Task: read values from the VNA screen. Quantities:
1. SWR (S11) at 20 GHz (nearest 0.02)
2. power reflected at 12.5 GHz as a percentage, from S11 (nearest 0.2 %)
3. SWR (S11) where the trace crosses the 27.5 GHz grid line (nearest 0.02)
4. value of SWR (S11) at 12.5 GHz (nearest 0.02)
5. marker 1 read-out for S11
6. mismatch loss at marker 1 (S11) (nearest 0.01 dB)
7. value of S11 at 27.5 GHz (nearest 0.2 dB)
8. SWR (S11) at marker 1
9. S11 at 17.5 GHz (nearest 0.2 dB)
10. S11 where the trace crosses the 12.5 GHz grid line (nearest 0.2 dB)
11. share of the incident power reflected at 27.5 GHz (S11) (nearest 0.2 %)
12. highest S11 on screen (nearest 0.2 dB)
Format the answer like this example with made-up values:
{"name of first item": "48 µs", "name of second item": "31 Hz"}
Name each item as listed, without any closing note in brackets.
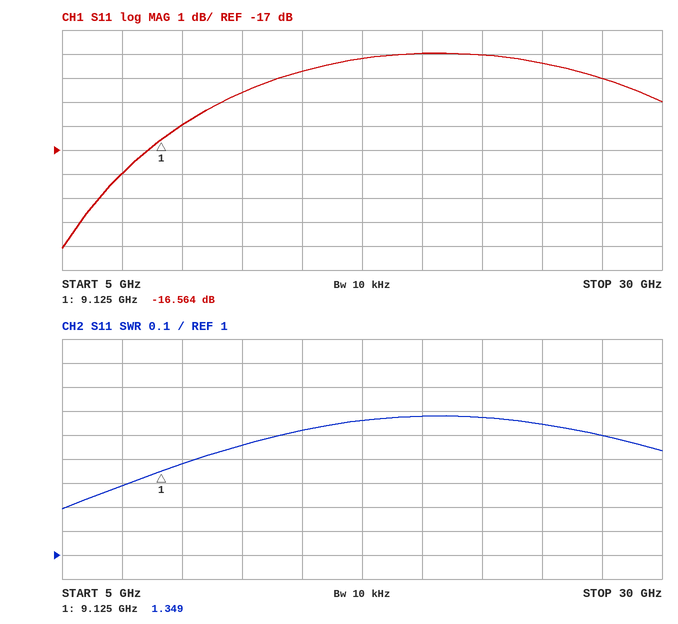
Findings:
{"SWR (S11) at 20 GHz": "1.58", "power reflected at 12.5 GHz as a percentage, from S11": "3.4 %", "SWR (S11) where the trace crosses the 27.5 GHz grid line": "1.50", "value of SWR (S11) at 12.5 GHz": "1.46", "marker 1 read-out for S11": "-16.564 dB", "mismatch loss at marker 1 (S11)": "0.10 dB", "value of S11 at 27.5 GHz": "-14.0 dB", "SWR (S11) at marker 1": "1.349", "S11 at 17.5 GHz": "-13.2 dB", "S11 where the trace crosses the 12.5 GHz grid line": "-14.6 dB", "share of the incident power reflected at 27.5 GHz (S11)": "4.0 %", "highest S11 on screen": "-13.0 dB"}
